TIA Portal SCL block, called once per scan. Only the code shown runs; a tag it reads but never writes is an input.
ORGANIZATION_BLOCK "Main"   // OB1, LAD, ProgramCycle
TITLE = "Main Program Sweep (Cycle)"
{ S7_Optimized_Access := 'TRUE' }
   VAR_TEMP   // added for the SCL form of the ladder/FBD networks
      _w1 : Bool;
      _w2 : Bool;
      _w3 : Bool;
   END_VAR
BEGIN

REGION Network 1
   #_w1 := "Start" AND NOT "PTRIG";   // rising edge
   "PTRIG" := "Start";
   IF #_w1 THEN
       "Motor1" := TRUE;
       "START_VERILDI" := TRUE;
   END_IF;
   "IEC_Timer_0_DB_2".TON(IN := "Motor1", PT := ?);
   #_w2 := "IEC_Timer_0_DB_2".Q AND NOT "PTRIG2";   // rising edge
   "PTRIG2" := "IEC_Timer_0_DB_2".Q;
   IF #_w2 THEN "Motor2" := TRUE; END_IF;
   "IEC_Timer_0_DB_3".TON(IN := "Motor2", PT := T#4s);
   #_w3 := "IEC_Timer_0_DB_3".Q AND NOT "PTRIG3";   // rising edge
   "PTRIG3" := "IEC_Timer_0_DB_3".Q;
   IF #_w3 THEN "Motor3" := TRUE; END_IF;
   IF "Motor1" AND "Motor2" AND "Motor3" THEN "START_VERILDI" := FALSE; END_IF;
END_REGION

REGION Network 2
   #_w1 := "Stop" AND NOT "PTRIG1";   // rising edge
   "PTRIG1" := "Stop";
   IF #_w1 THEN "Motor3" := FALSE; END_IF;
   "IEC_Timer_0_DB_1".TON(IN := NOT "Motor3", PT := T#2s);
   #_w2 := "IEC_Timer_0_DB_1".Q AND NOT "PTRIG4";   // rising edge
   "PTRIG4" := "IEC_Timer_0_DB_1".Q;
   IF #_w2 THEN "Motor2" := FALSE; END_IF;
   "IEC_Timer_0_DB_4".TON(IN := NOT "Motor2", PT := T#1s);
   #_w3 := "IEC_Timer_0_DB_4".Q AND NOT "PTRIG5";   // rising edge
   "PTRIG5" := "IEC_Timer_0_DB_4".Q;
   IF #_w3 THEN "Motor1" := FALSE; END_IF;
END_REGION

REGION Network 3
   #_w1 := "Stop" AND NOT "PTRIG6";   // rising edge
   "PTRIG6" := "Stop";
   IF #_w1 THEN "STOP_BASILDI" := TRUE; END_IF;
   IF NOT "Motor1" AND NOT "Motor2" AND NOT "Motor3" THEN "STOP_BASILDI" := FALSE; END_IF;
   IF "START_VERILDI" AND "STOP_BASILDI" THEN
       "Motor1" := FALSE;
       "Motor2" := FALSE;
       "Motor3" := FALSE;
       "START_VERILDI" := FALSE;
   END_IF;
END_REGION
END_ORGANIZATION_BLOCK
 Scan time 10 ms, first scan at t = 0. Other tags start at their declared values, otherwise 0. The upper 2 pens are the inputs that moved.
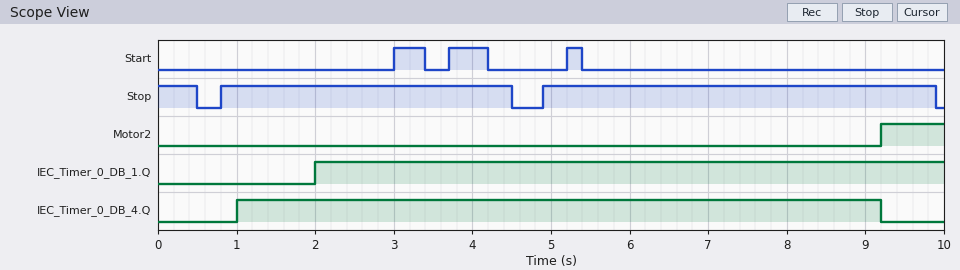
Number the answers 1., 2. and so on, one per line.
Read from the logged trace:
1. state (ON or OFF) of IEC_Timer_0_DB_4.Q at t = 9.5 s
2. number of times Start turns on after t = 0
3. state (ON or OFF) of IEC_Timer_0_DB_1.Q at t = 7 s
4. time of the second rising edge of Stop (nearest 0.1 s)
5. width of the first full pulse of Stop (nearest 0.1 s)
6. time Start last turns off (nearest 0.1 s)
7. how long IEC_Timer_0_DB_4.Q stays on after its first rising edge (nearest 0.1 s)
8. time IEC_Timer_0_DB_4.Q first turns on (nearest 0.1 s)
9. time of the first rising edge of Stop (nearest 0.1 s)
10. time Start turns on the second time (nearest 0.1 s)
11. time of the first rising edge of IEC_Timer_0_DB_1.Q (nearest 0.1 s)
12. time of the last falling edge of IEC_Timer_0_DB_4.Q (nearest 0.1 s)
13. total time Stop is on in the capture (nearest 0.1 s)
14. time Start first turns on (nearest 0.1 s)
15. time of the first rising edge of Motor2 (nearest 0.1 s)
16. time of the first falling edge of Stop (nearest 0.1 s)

1. OFF
2. 3
3. ON
4. 4.9 s
5. 3.7 s
6. 5.4 s
7. 8.2 s
8. 1.0 s
9. 0.8 s
10. 3.7 s
11. 2.0 s
12. 9.2 s
13. 9.2 s
14. 3.0 s
15. 9.2 s
16. 0.5 s
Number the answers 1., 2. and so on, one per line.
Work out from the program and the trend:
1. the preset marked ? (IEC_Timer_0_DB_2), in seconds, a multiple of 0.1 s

1. 4.0 s
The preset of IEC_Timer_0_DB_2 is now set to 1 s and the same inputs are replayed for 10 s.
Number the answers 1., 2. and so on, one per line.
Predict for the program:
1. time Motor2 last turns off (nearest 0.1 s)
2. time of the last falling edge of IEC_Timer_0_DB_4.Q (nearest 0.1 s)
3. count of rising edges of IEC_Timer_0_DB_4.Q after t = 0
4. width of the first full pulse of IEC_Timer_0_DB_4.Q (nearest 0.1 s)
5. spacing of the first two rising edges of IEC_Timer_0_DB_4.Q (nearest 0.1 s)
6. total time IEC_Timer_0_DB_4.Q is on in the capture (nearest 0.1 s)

1. 4.9 s
2. 4.0 s
3. 2
4. 3.0 s
5. 4.9 s
6. 7.1 s
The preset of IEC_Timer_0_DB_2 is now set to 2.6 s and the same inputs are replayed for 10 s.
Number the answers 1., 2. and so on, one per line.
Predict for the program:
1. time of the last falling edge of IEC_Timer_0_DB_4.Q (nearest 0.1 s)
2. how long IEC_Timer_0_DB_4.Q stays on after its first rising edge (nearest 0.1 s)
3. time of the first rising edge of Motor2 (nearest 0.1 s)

1. 7.8 s
2. 6.8 s
3. 7.8 s
